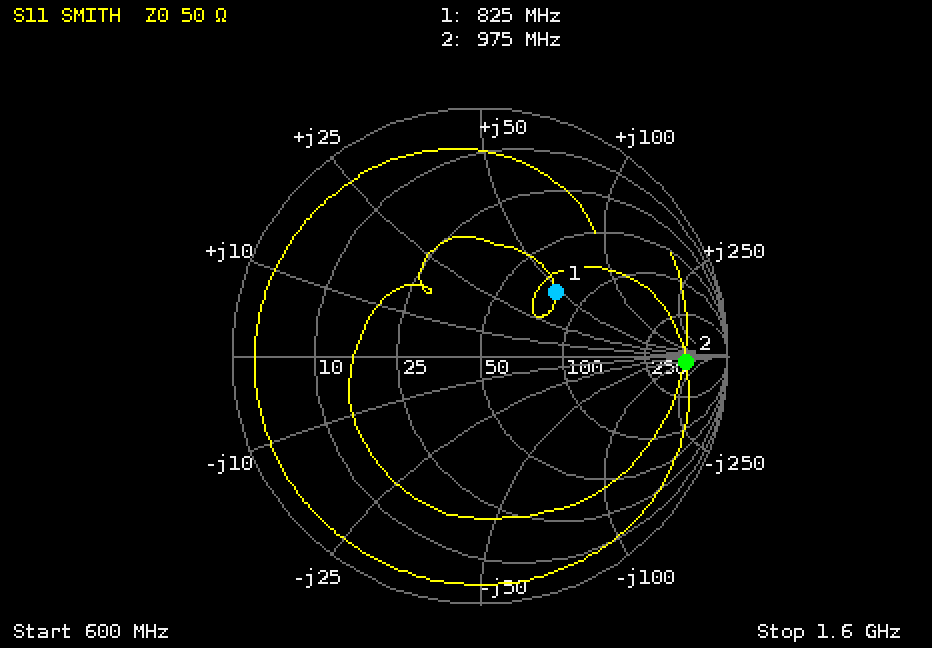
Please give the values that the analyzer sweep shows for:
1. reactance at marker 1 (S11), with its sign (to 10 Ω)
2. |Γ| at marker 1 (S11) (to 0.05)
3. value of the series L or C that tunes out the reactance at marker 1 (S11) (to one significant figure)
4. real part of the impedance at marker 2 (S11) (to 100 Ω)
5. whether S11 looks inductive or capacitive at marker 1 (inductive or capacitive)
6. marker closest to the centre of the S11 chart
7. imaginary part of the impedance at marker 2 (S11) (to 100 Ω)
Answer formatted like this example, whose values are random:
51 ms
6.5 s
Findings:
+50 Ω
0.40
4 pF
500 Ω
inductive
marker 1
-100 Ω
